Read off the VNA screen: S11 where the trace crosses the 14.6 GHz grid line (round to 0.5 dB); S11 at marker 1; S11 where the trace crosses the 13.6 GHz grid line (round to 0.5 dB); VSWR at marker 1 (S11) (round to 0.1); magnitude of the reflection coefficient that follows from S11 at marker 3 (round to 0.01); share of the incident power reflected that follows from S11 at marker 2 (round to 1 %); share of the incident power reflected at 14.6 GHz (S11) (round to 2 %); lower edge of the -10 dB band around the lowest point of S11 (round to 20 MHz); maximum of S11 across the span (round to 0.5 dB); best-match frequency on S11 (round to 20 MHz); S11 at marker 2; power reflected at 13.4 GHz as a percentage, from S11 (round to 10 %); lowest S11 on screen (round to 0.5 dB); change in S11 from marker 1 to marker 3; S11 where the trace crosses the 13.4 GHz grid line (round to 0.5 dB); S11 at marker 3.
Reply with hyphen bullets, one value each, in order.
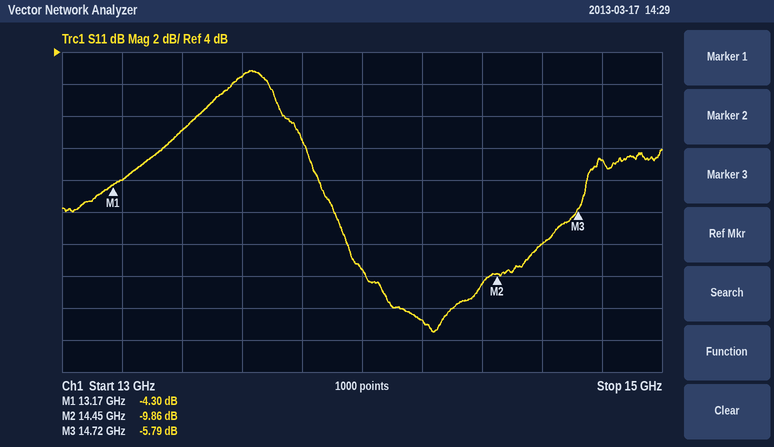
- -8.0 dB
- -4.30 dB
- 2.5 dB
- 4.1
- 0.51
- 10 %
- 16 %
- 14.02 GHz
- 3.0 dB
- 14.24 GHz
- -9.86 dB
- 80 %
- -13.5 dB
- -1.49 dB
- -1.0 dB
- -5.79 dB
